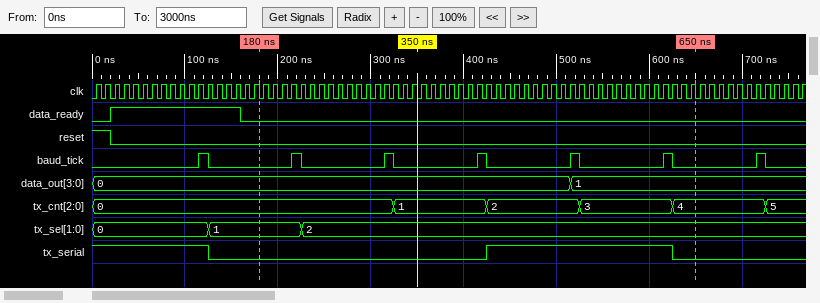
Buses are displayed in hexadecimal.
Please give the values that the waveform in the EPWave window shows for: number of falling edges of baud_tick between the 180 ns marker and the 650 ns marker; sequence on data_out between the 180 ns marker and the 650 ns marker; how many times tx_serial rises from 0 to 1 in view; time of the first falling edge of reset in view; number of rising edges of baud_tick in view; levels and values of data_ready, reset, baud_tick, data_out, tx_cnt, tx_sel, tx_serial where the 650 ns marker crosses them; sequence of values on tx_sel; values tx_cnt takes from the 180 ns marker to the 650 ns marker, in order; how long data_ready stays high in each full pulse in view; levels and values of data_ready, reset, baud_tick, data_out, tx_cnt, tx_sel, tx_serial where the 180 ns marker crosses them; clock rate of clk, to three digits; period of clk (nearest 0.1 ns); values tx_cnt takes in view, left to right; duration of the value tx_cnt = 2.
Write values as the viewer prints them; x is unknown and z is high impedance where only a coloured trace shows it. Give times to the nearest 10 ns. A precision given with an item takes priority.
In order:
5
0, 1
1
20 ns
7
data_ready=0, reset=0, baud_tick=0, data_out=1, tx_cnt=4, tx_sel=2, tx_serial=0
0, 1, 2
0, 1, 2, 3, 4
140 ns
data_ready=0, reset=0, baud_tick=0, data_out=0, tx_cnt=0, tx_sel=1, tx_serial=0
100 MHz
10 ns
0, 1, 2, 3, 4, 5
100 ns
